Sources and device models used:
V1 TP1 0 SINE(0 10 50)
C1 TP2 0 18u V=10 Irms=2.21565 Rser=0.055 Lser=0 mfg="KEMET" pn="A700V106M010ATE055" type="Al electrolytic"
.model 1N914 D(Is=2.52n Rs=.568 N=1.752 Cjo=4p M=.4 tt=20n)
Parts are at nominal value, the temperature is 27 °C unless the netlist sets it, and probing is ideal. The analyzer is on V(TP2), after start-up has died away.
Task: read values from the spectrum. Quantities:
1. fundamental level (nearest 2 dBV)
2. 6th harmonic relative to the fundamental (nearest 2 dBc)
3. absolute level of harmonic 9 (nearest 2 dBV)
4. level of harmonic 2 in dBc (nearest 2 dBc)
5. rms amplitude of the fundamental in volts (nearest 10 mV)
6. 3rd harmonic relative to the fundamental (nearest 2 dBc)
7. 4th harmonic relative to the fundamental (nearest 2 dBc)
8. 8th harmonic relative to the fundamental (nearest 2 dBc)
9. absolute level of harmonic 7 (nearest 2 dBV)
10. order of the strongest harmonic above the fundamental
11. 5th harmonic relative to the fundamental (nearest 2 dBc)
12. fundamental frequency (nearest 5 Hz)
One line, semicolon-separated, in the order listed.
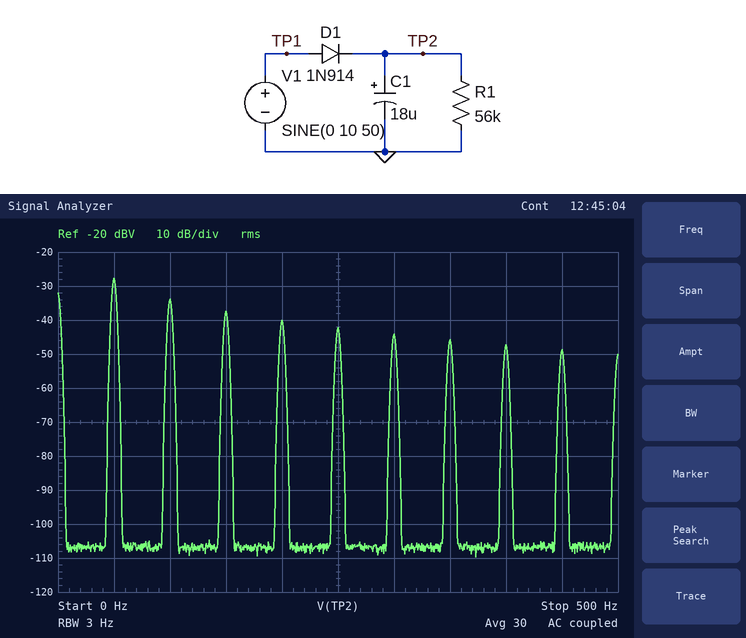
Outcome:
-28 dBV; -16 dBc; -48 dBV; -6 dBc; 40 mV; -10 dBc; -12 dBc; -20 dBc; -46 dBV; 2; -14 dBc; 50 Hz
